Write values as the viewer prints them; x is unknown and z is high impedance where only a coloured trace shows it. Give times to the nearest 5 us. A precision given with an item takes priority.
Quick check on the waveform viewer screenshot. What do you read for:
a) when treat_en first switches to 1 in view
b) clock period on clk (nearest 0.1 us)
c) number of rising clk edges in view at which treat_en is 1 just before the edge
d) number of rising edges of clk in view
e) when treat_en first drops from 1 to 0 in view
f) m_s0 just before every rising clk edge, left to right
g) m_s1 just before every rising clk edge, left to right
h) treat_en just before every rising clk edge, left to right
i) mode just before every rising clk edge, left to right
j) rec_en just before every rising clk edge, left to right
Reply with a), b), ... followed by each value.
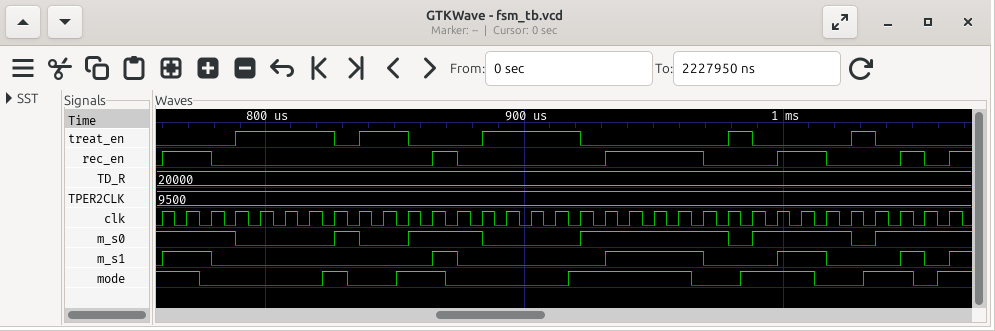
a) 790 us
b) 9.5 us
c) 12
d) 33
e) 825 us
f) 1 1 1 1 0 0 0 0 1 0 0 1 1 1 0 0 0 0 1 1 1 1 1 1 0 1 1 1 1 0 1 1 1
g) 0 1 1 0 0 0 0 0 0 0 0 0 1 0 0 0 0 0 0 1 1 1 1 0 0 0 1 1 0 0 0 1 0
h) 0 0 0 0 1 1 1 1 0 1 1 0 0 0 1 1 1 1 0 0 0 0 0 0 1 0 0 0 0 1 0 0 0
i) 1 1 0 0 0 0 0 1 0 0 1 1 0 0 0 0 0 1 1 1 1 1 0 0 1 1 1 0 0 1 1 0 1
j) 0 1 1 0 0 0 0 0 0 0 0 0 1 0 0 0 0 0 0 1 1 1 1 0 0 0 1 1 0 0 0 1 0
